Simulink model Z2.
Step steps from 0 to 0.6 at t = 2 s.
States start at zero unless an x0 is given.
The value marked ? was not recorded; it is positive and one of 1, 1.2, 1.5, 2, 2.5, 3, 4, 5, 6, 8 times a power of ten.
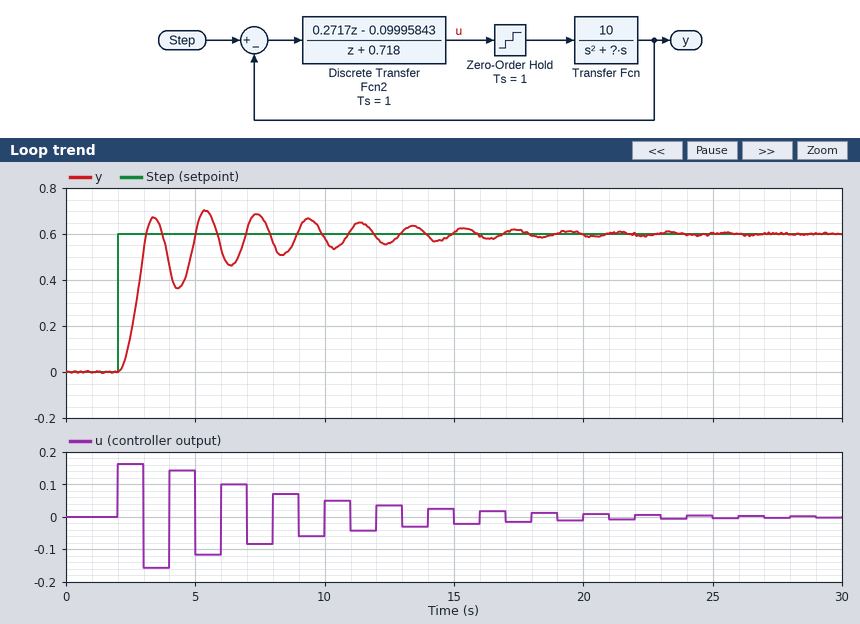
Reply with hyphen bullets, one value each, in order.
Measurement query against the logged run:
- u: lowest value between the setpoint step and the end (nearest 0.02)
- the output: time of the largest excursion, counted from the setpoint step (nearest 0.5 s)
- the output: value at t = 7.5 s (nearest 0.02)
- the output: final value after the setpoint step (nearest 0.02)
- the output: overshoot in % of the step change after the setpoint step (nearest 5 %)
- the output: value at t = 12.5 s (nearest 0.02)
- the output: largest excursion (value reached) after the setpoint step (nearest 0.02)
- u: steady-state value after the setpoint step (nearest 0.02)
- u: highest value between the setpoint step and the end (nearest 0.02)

- -0.16
- 3.5 s
- 0.68
- 0.60
- 15 %
- 0.56
- 0.70
- 0.00
- 0.16
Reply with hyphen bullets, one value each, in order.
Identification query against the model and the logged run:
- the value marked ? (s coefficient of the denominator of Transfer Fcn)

- 1.5
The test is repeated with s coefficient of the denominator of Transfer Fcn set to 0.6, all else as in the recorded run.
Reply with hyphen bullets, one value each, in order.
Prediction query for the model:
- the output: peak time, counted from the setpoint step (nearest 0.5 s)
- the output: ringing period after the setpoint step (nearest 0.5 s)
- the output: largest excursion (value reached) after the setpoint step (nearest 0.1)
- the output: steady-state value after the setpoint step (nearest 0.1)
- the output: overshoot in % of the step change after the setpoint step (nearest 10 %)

- 1.5 s
- 2.0 s
- 1.0
- 0.6
- 60 %
